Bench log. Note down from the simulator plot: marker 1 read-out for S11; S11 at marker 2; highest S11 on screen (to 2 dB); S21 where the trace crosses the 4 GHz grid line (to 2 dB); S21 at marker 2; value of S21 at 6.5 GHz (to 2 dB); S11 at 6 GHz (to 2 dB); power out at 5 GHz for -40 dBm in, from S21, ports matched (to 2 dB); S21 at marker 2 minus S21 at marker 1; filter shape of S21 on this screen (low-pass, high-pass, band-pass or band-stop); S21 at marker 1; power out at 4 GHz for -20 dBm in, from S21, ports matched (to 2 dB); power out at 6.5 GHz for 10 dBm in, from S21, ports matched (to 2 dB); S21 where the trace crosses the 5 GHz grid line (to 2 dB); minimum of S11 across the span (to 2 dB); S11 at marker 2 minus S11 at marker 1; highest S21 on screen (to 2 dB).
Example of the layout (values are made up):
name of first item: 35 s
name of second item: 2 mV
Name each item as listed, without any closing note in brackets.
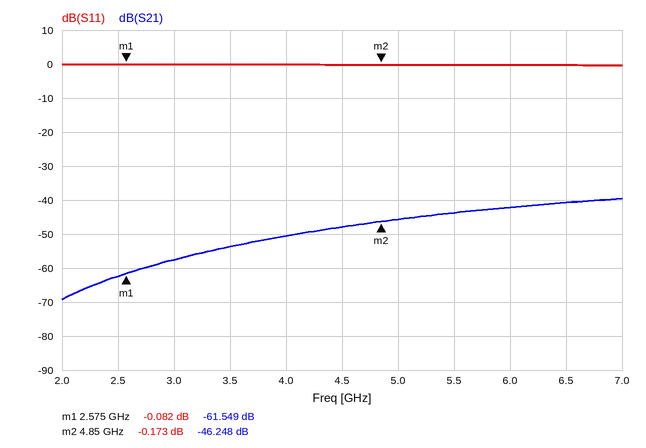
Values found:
marker 1 read-out for S11: -0.082 dB
S11 at marker 2: -0.173 dB
highest S11 on screen: 0 dB
S21 where the trace crosses the 4 GHz grid line: -50 dB
S21 at marker 2: -46.248 dB
value of S21 at 6.5 GHz: -40 dB
S11 at 6 GHz: 0 dB
power out at 5 GHz for -40 dBm in, from S21, ports matched: -86 dBm
S21 at marker 2 minus S21 at marker 1: 15.301 dB
filter shape of S21 on this screen: high-pass
S21 at marker 1: -61.549 dB
power out at 4 GHz for -20 dBm in, from S21, ports matched: -70 dBm
power out at 6.5 GHz for 10 dBm in, from S21, ports matched: -30 dBm
S21 where the trace crosses the 5 GHz grid line: -46 dB
minimum of S11 across the span: 0 dB
S11 at marker 2 minus S11 at marker 1: -0.091 dB
highest S21 on screen: -40 dB
